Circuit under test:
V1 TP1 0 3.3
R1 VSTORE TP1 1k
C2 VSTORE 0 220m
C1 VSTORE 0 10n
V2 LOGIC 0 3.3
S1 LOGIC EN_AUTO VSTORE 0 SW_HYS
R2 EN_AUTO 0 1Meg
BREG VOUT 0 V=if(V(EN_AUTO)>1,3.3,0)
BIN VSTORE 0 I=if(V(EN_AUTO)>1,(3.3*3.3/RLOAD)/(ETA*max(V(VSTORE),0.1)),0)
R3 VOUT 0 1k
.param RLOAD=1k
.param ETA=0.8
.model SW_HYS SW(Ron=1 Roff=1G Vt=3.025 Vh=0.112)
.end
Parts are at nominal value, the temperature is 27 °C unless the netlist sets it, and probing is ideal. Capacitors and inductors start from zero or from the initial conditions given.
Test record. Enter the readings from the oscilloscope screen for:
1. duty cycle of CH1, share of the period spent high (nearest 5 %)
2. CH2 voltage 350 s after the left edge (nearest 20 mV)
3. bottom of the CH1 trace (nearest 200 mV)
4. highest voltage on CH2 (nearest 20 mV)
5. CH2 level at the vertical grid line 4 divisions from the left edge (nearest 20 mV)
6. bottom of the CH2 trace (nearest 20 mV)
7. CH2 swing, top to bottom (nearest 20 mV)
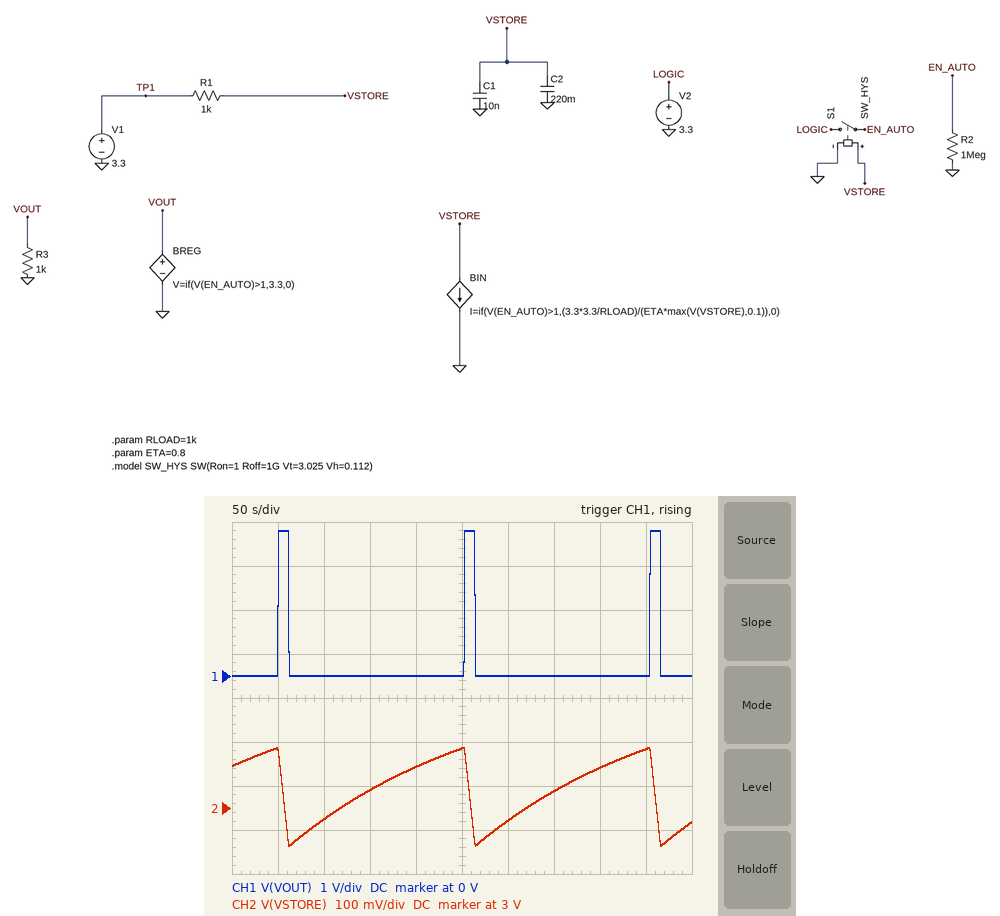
5 %
3.04 V
0 V
3.14 V
3.10 V
2.92 V
220 mV
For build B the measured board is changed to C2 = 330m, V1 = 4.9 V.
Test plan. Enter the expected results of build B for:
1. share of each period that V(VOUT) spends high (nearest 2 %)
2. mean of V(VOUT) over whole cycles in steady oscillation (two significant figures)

42 %
1.4 V
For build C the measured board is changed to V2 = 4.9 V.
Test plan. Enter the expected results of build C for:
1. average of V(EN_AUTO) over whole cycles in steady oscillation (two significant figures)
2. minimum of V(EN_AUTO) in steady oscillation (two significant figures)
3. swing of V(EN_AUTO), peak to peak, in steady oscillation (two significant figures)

290 mV
4.9 mV
4.9 V
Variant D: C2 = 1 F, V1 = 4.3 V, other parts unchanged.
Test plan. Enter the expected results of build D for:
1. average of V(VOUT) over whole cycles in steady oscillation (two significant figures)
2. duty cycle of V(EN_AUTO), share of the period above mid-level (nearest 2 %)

930 mV
28 %
